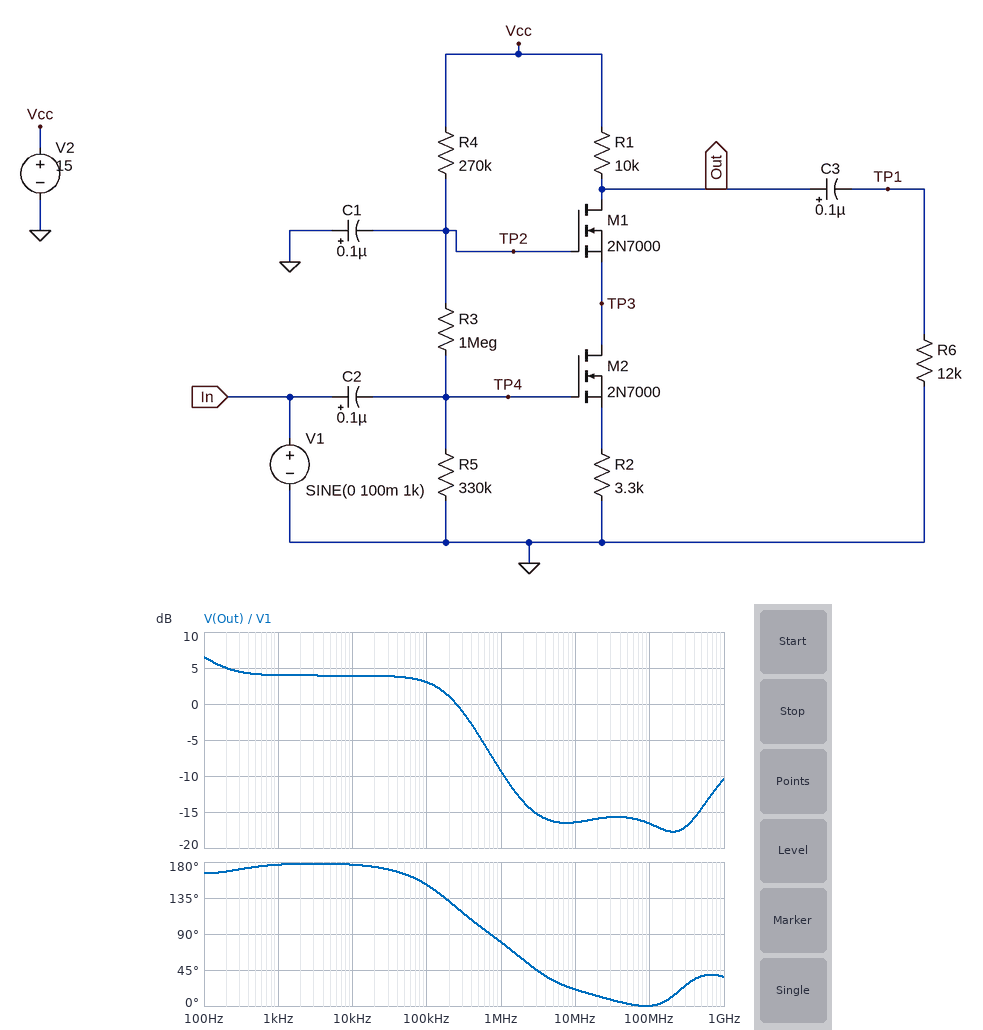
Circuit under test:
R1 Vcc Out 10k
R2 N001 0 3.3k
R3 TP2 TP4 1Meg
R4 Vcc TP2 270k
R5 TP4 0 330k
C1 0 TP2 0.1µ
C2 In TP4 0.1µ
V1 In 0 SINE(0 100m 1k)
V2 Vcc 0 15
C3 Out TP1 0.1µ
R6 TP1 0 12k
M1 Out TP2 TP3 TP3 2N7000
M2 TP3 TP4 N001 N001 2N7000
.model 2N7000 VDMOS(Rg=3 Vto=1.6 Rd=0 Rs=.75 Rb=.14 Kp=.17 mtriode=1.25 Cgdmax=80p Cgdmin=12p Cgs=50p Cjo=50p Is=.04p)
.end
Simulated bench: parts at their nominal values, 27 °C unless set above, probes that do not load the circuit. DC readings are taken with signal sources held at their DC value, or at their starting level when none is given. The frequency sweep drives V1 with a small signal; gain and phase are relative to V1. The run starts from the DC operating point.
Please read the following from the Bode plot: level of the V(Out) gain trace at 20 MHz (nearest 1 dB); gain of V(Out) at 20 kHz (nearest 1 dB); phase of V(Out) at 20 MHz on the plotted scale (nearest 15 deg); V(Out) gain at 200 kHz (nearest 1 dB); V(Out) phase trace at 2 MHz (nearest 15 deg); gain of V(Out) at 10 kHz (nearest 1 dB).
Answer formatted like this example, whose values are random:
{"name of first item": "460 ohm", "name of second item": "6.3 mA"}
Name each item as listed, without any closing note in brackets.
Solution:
{"level of the V(Out) gain trace at 20 MHz": "-16 dB", "gain of V(Out) at 20 kHz": "4 dB", "phase of V(Out) at 20 MHz on the plotted scale": "15 deg", "V(Out) gain at 200 kHz": "1 dB", "V(Out) phase trace at 2 MHz": "60 deg", "gain of V(Out) at 10 kHz": "4 dB"}
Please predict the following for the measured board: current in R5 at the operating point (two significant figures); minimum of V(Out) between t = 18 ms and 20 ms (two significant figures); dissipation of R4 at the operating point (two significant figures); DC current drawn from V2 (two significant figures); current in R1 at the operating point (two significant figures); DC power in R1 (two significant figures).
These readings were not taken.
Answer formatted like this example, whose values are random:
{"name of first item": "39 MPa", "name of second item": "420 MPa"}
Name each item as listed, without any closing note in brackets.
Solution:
{"current in R5 at the operating point": "9.4 µA", "minimum of V(Out) between t = 18 ms and 20 ms": "10 V", "dissipation of R4 at the operating point": "24 µW", "DC current drawn from V2": "460 µA", "current in R1 at the operating point": "450 µA", "DC power in R1": "2.0 mW"}
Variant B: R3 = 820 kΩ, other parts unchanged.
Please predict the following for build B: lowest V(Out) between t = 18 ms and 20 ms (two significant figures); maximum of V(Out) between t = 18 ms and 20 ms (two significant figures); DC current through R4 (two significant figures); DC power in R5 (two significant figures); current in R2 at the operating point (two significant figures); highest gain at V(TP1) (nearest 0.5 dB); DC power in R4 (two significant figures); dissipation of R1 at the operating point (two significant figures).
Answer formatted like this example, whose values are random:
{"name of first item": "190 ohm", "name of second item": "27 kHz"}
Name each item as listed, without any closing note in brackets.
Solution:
{"lowest V(Out) between t = 18 ms and 20 ms": "9.2 V", "maximum of V(Out) between t = 18 ms and 20 ms": "9.5 V", "DC current through R4": "11 µA", "DC power in R5": "37 µW", "current in R2 at the operating point": "560 µA", "highest gain at V(TP1)": "4.0 dB", "DC power in R4": "30 µW", "dissipation of R1 at the operating point": "3.2 mW"}
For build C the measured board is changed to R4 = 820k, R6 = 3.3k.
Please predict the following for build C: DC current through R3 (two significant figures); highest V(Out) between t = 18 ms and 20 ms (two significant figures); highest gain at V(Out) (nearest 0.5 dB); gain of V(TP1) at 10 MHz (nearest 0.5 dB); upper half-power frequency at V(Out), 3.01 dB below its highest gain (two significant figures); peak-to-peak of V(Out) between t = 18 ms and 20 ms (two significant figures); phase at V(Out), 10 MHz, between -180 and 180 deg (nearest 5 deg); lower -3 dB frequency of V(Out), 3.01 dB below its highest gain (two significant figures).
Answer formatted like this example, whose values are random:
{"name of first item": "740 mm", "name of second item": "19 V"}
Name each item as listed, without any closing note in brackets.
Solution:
{"DC current through R3": "7.0 µA", "highest V(Out) between t = 18 ms and 20 ms": "13 V", "highest gain at V(Out)": "8.5 dB", "gain of V(TP1) at 10 MHz": "-6.0 dB", "upper half-power frequency at V(Out), 3.01 dB below its highest gain": "140 Hz", "peak-to-peak of V(Out) between t = 18 ms and 20 ms": "150 mV", "phase at V(Out), 10 MHz, between -180 and 180 deg": "-25 deg", "lower -3 dB frequency of V(Out), 3.01 dB below its highest gain": "5.9 Hz"}
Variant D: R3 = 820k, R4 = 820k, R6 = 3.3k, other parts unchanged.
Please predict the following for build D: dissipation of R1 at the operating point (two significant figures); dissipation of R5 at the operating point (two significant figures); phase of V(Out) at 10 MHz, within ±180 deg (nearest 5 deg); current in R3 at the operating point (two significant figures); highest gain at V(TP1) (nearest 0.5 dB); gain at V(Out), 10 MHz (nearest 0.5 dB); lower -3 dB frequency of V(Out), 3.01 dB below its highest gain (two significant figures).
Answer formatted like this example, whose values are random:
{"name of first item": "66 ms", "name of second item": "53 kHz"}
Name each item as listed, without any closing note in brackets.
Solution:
{"dissipation of R1 at the operating point": "810 µW", "dissipation of R5 at the operating point": "19 µW", "phase of V(Out) at 10 MHz, within ±180 deg": "-25 deg", "current in R3 at the operating point": "7.6 µA", "highest gain at V(TP1)": "0 dB", "gain at V(Out), 10 MHz": "-4.5 dB", "lower -3 dB frequency of V(Out), 3.01 dB below its highest gain": "6.2 Hz"}
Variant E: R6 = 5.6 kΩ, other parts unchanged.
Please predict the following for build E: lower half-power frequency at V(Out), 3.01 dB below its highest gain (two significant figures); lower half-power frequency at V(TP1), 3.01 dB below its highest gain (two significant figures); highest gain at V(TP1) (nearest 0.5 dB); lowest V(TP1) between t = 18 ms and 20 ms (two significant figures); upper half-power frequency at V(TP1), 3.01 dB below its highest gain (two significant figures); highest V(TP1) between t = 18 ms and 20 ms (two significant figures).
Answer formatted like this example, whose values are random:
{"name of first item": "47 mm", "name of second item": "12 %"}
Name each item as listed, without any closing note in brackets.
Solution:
{"lower half-power frequency at V(Out), 3.01 dB below its highest gain": "5.7 Hz", "lower half-power frequency at V(TP1), 3.01 dB below its highest gain": "100 Hz", "highest gain at V(TP1)": "0.5 dB", "lowest V(TP1) between t = 18 ms and 20 ms": "-100 mV", "upper half-power frequency at V(TP1), 3.01 dB below its highest gain": "310 kHz", "highest V(TP1) between t = 18 ms and 20 ms": "100 mV"}
